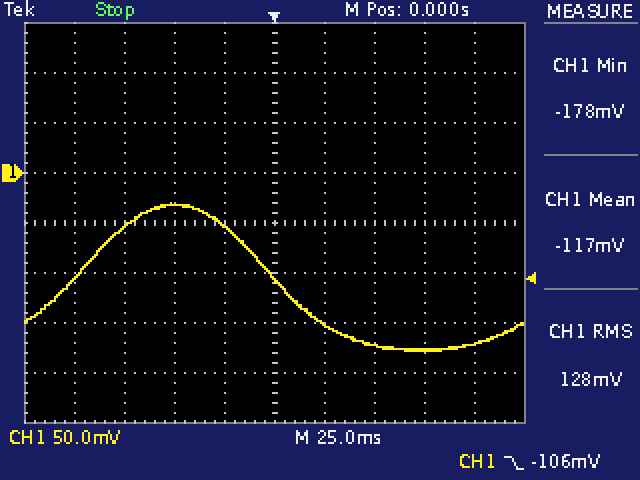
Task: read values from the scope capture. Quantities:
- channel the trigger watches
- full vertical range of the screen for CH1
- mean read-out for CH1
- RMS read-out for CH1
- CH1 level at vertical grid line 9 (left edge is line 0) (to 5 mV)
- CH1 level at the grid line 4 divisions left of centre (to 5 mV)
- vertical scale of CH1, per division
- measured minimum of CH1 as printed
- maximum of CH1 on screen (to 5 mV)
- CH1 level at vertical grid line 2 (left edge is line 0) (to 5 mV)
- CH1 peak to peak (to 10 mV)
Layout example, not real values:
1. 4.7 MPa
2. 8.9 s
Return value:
1. CH1
2. 400 mV
3. -117 mV
4. 128 mV
5. -170 mV
6. -105 mV
7. 50 mV
8. -178 mV
9. -30 mV
10. -55 mV
11. 150 mV
